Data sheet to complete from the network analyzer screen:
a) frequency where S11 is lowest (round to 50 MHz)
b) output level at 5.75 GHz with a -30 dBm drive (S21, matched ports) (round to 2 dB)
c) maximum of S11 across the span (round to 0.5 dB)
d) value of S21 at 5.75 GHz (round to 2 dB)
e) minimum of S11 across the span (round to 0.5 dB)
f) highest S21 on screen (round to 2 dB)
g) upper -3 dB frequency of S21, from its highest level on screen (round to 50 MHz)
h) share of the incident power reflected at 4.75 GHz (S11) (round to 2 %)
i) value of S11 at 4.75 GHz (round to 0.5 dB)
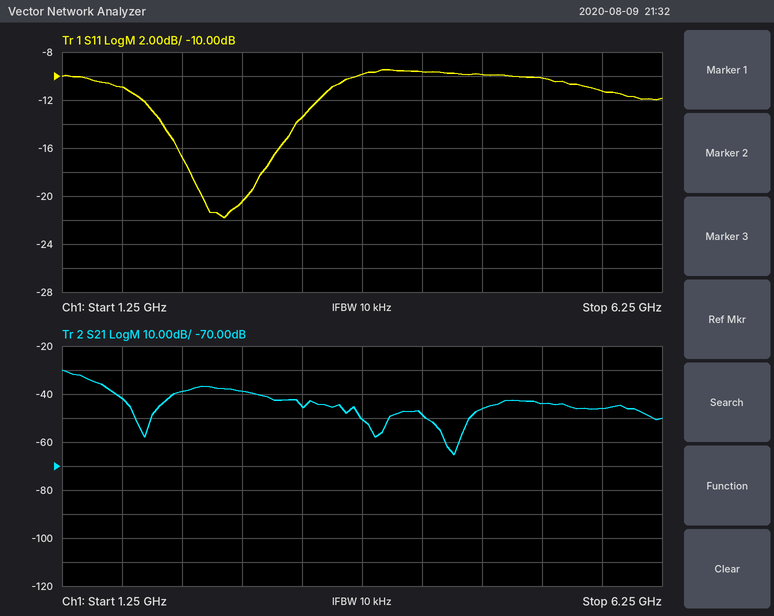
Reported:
2.60 GHz
-76 dBm
-9.5 dB
-46 dB
-22.0 dB
-30 dB
1.45 GHz
10 %
-10.0 dB
